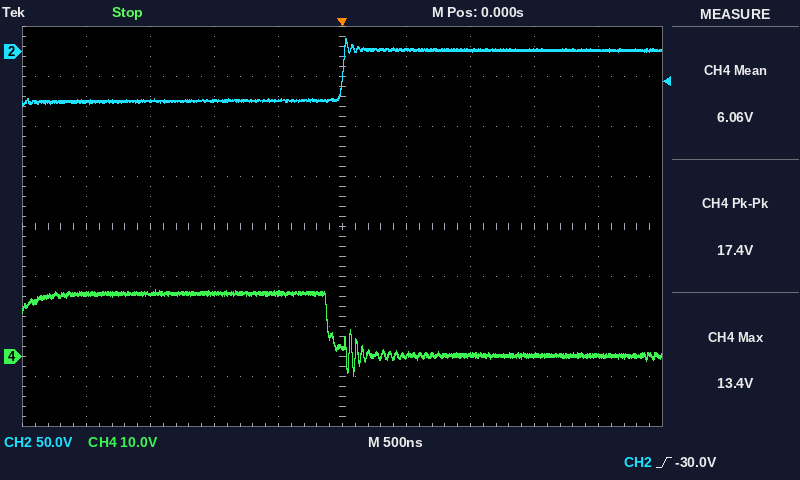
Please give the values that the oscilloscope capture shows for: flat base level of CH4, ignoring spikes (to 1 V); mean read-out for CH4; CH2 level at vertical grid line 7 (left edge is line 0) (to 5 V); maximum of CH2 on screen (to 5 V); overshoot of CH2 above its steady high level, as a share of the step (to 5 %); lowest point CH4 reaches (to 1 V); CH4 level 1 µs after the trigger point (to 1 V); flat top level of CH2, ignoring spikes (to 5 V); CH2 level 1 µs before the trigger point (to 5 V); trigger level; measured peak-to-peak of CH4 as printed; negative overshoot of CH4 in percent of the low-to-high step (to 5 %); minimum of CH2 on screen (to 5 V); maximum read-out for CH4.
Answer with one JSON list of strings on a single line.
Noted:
["0 V", "6.06 V", "0 V", "15 V", "25 %", "-4 V", "0 V", "0 V", "-50 V", "-30.0 V", "17.4 V", "35 %", "-55 V", "13.4 V"]
